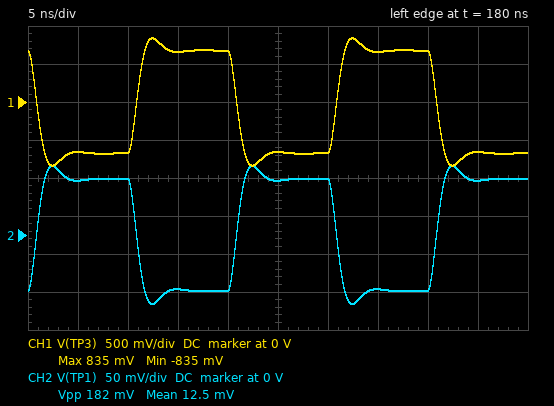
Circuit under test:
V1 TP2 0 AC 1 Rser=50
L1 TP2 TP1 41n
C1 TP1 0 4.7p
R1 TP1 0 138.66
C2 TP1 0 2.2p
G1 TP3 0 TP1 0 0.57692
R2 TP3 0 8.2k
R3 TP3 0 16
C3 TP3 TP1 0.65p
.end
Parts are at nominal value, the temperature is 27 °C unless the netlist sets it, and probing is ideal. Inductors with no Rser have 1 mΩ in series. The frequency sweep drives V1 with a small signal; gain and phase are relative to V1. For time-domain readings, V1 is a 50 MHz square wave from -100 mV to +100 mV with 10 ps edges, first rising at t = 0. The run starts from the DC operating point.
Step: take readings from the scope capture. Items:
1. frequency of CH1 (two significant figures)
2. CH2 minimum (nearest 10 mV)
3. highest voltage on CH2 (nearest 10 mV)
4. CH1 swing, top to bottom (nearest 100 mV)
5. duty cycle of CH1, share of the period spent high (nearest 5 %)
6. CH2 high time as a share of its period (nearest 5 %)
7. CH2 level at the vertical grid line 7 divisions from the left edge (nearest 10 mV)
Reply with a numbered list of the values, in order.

1. 50 MHz
2. -90 mV
3. 90 mV
4. 1.7 V
5. 50 %
6. 50 %
7. -70 mV
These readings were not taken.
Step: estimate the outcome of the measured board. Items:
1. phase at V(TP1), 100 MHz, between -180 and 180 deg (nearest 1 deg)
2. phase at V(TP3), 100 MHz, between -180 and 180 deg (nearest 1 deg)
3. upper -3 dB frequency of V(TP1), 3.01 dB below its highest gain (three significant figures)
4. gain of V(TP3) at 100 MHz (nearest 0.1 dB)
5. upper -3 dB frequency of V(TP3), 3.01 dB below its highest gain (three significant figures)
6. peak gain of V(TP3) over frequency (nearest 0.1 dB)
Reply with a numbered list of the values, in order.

1. -28 deg
2. 151 deg
3. 283 MHz
4. 17.0 dB
5. 283 MHz
6. 17.2 dB
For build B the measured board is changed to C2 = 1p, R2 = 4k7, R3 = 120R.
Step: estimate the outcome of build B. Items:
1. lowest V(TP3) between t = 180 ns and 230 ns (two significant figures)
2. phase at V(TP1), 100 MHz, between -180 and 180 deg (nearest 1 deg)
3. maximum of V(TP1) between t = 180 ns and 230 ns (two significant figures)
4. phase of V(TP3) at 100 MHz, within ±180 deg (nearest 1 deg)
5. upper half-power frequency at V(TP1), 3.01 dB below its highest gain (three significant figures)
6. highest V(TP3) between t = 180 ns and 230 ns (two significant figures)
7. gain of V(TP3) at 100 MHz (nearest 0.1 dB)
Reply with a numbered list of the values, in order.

1. -5.0 V
2. -71 deg
3. 74 mV
4. 106 deg
5. 102 MHz
6. 5.0 V
7. 31.0 dB
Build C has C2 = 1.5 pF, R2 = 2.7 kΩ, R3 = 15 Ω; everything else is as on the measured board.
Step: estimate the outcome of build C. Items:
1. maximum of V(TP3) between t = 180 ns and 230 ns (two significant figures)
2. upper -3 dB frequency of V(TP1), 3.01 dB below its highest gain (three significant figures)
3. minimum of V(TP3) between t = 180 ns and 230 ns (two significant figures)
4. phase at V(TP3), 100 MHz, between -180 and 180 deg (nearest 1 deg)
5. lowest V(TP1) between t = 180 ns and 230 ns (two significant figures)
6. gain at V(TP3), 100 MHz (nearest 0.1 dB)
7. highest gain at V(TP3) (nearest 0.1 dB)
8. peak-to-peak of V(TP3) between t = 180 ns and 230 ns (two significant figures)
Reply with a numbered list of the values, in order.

1. 790 mV
2. 297 MHz
3. -790 mV
4. 153 deg
5. -92 mV
6. 16.4 dB
7. 16.7 dB
8. 1.6 V
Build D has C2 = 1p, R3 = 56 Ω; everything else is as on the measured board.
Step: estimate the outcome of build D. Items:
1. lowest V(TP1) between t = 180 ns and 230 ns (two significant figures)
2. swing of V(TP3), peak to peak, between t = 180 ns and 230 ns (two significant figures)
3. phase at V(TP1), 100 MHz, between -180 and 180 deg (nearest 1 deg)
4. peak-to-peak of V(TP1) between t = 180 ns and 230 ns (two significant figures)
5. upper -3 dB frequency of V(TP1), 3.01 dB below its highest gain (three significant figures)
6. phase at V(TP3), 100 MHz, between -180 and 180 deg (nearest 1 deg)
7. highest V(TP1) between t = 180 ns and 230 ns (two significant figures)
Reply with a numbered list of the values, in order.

1. -81 mV
2. 5.2 V
3. -48 deg
4. 160 mV
5. 180 MHz
6. 130 deg
7. 81 mV
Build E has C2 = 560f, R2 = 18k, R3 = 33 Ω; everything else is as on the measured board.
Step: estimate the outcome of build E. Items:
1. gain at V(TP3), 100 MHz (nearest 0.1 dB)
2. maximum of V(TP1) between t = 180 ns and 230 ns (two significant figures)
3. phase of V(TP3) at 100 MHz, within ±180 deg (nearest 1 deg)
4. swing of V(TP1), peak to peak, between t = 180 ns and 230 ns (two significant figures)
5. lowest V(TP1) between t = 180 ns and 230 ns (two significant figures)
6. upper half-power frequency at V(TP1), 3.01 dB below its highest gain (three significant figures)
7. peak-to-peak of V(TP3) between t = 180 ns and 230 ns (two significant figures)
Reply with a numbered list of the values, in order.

1. 23.2 dB
2. 87 mV
3. 144 deg
4. 170 mV
5. -87 mV
6. 237 MHz
7. 3.3 V
